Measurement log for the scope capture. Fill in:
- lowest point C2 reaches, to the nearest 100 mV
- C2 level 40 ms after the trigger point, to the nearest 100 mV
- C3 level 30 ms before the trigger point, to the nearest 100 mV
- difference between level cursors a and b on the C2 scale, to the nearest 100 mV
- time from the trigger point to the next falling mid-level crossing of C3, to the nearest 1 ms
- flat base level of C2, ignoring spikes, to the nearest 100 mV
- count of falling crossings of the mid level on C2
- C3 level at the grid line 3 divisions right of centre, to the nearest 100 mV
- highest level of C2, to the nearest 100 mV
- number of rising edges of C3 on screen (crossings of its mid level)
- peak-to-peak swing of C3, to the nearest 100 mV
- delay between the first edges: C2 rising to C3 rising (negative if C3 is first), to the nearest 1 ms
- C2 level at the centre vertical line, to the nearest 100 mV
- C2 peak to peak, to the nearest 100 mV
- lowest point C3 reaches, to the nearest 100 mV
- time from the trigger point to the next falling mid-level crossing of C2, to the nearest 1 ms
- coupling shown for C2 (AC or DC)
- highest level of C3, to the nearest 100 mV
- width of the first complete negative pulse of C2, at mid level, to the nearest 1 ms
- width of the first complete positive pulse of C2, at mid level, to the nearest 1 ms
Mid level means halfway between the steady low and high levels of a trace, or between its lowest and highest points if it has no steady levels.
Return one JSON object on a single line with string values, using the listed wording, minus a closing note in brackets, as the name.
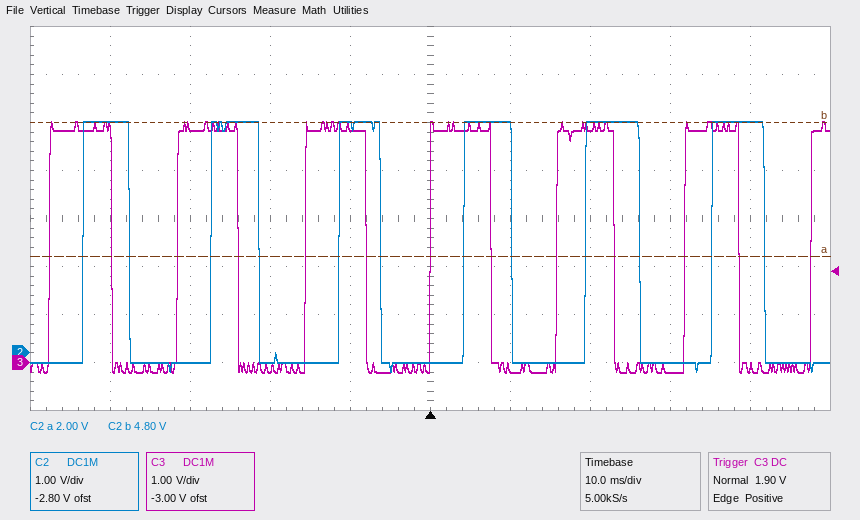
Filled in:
{"lowest point C2 reaches, to the nearest 100 mV": "-400 mV", "C2 level 40 ms after the trigger point, to the nearest 100 mV": "4.8 V", "C3 level 30 ms before the trigger point, to the nearest 100 mV": "4.9 V", "difference between level cursors a and b on the C2 scale, to the nearest 100 mV": "2.8 V", "time from the trigger point to the next falling mid-level crossing of C3, to the nearest 1 ms": "8 ms", "flat base level of C2, ignoring spikes, to the nearest 100 mV": "-200 mV", "count of falling crossings of the mid level on C2": "6", "C3 level at the grid line 3 divisions right of centre, to the nearest 100 mV": "-200 mV", "highest level of C2, to the nearest 100 mV": "4.8 V", "number of rising edges of C3 on screen": "7", "peak-to-peak swing of C3, to the nearest 100 mV": "5.2 V", "delay between the first edges: C2 rising to C3 rising (negative if C3 is first), to the nearest 1 ms": "-4 ms", "C2 level at the centre vertical line, to the nearest 100 mV": "-200 mV", "C2 peak to peak, to the nearest 100 mV": "5.2 V", "lowest point C3 reaches, to the nearest 100 mV": "-200 mV", "time from the trigger point to the next falling mid-level crossing of C2, to the nearest 1 ms": "10 ms", "coupling shown for C2": "DC", "highest level of C3, to the nearest 100 mV": "5.0 V", "width of the first complete negative pulse of C2, at mid level, to the nearest 1 ms": "10 ms", "width of the first complete positive pulse of C2, at mid level, to the nearest 1 ms": "6 ms"}
